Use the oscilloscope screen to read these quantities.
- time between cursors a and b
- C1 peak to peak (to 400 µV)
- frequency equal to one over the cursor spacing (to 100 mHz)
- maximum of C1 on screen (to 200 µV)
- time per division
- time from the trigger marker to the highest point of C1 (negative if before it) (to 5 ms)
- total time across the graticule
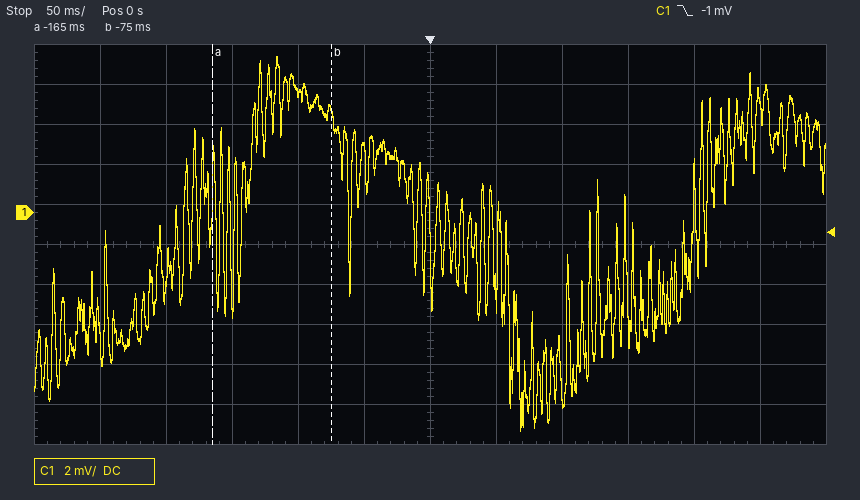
90 ms
18.8 mV
11.1 Hz
7.8 mV
50 ms
-115 ms
600 ms
